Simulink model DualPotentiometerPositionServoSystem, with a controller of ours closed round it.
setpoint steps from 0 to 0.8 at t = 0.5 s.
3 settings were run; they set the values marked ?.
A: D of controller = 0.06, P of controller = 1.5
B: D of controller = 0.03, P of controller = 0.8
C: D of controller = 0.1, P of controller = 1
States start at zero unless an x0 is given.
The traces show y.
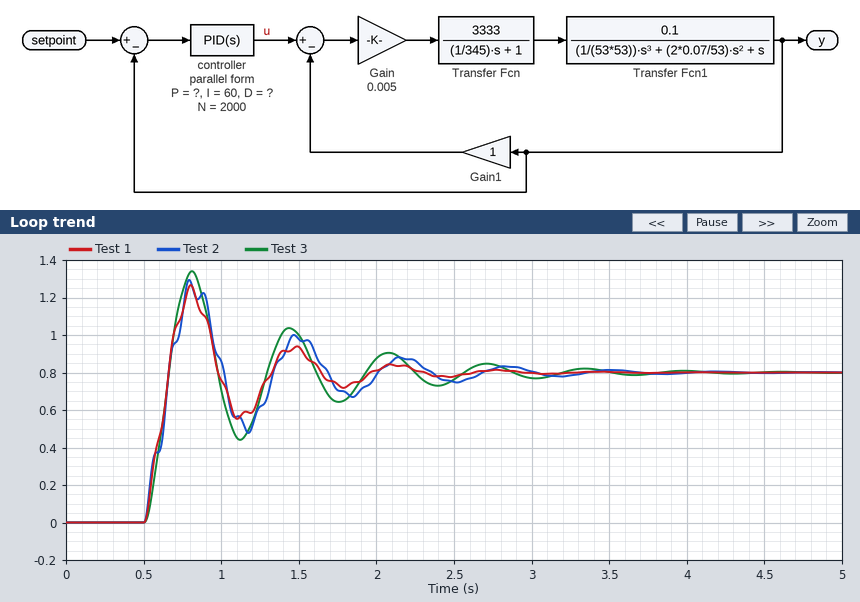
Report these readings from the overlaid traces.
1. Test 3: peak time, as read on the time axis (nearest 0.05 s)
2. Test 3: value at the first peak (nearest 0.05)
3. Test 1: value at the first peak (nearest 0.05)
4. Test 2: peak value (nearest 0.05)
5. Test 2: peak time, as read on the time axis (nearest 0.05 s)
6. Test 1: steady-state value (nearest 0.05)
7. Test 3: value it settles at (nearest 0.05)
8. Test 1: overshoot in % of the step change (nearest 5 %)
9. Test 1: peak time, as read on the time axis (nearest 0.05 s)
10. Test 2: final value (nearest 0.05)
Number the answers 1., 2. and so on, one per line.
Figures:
1. 0.80 s
2. 1.35
3. 1.25
4. 1.30
5. 0.80 s
6. 0.80
7. 0.80
8. 60 %
9. 0.80 s
10. 0.80
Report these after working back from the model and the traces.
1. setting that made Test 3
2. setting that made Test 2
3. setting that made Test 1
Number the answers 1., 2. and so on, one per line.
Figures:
1. B
2. C
3. A
